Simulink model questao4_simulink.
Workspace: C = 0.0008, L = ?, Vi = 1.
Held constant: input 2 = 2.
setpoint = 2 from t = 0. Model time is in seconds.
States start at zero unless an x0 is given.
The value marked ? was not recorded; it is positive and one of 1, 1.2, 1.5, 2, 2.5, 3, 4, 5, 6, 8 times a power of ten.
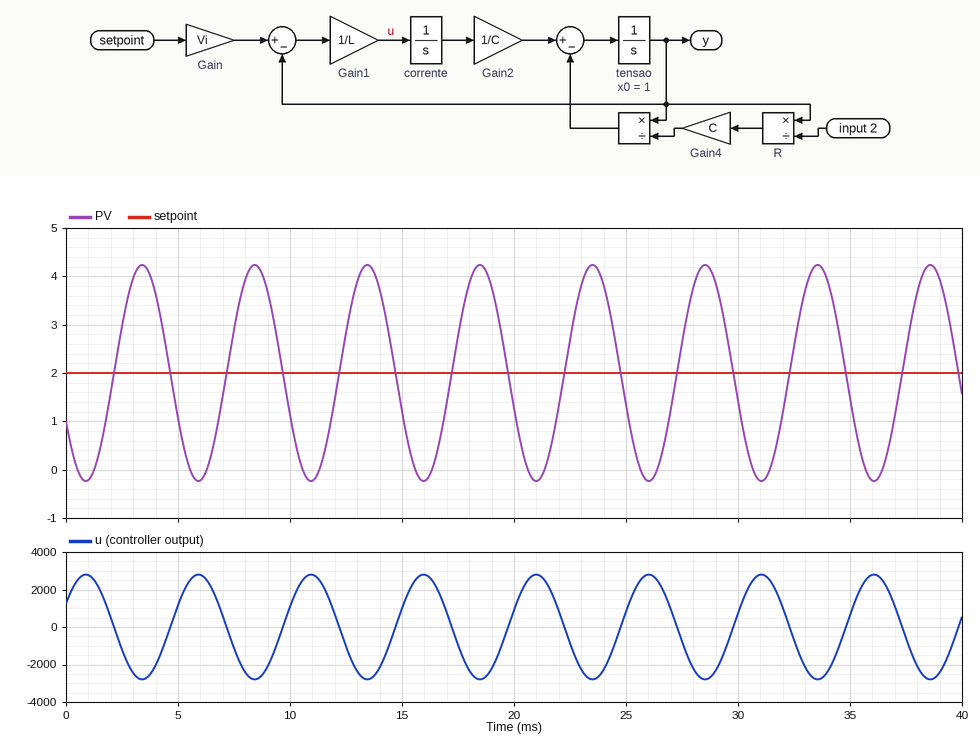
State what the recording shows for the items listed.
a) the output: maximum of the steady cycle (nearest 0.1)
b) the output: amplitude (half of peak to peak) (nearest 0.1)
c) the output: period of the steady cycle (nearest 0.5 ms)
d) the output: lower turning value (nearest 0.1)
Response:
4.2
2.2
5.0 ms
-0.2
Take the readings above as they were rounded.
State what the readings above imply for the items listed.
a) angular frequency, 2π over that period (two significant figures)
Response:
1.3 rad/ms
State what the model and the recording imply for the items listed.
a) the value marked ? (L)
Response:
0.0008
